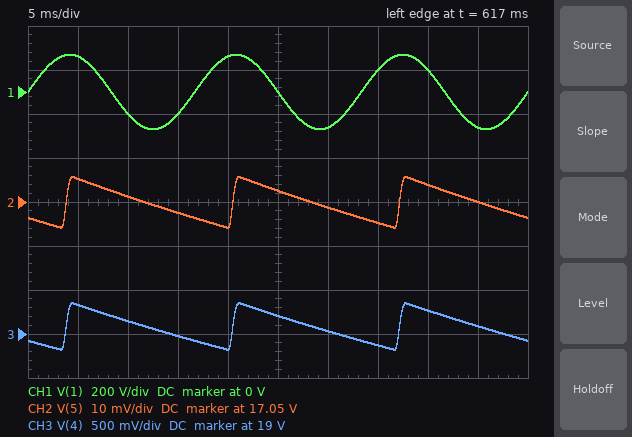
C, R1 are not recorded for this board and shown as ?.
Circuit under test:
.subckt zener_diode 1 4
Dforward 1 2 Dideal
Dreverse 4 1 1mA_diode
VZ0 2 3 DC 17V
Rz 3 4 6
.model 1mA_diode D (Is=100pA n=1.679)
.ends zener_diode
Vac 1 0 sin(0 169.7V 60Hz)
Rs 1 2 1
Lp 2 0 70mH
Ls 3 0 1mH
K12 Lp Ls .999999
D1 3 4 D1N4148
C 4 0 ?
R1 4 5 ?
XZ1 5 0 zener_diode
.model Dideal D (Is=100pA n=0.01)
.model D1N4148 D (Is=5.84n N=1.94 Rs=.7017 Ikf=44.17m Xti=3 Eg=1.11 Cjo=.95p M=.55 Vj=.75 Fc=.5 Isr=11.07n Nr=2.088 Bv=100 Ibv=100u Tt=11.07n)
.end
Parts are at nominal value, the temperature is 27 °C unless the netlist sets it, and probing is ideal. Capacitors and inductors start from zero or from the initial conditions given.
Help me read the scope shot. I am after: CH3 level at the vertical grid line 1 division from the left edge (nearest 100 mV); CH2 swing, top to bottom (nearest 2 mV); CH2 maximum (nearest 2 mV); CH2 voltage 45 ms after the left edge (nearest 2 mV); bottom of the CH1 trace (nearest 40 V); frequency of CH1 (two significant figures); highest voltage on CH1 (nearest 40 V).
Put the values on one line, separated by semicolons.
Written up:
19.3 V; 12 mV; 17.056 V; 17.050 V; -160 V; 60 Hz; 160 V
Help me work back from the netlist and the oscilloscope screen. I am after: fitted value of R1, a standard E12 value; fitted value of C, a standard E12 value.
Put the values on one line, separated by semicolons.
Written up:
270 Ω; 220 µF
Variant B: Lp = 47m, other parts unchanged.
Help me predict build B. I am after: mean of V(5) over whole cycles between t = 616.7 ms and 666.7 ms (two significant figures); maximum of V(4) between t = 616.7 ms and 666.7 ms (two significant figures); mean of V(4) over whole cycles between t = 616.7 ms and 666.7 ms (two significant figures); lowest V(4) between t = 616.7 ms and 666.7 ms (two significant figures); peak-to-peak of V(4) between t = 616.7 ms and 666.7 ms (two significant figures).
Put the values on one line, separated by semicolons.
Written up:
17 V; 24 V; 23 V; 22 V; 1.5 V
